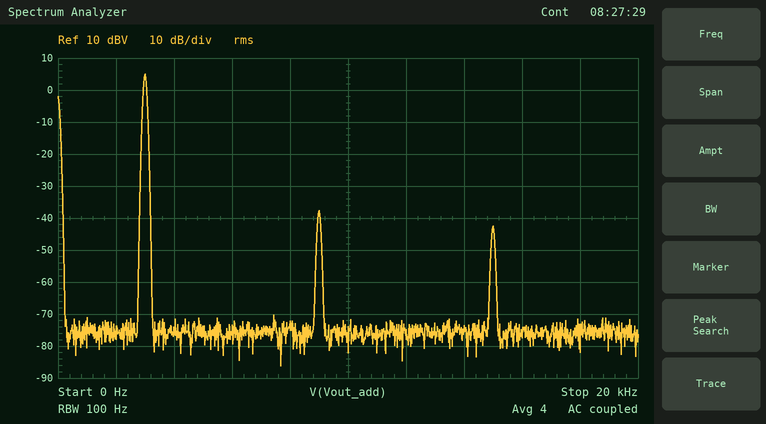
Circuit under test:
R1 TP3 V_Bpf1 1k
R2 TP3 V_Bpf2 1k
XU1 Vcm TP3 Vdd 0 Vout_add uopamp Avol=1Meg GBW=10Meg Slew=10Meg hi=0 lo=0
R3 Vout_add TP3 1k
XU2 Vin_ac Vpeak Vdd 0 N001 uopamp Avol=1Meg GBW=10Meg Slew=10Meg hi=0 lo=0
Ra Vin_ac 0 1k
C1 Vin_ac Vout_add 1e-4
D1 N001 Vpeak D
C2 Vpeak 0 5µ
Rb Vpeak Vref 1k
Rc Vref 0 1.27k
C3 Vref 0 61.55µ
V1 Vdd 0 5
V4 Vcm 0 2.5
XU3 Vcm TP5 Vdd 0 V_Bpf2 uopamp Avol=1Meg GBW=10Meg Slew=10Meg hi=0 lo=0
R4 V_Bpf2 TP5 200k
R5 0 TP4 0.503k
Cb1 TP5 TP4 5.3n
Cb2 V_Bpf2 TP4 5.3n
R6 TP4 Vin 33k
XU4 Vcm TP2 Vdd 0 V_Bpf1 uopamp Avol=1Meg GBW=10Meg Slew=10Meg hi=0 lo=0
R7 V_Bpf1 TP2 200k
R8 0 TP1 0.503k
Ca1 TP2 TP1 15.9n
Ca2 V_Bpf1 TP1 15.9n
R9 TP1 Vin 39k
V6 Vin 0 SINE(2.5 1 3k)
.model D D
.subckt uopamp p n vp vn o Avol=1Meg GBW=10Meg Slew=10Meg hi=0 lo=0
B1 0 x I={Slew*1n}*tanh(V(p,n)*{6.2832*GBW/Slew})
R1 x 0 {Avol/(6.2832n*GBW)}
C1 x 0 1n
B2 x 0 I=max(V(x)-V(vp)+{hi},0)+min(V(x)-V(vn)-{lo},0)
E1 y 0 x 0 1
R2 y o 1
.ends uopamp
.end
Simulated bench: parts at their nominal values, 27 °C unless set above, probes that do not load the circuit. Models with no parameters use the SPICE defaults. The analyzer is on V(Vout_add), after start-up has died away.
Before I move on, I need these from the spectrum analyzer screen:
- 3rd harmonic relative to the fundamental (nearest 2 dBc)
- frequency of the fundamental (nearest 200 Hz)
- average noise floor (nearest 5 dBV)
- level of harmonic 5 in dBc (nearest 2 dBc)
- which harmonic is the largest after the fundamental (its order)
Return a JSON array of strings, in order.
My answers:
["-42 dBc", "3.0 kHz", "-75 dBV", "-48 dBc", "3"]
